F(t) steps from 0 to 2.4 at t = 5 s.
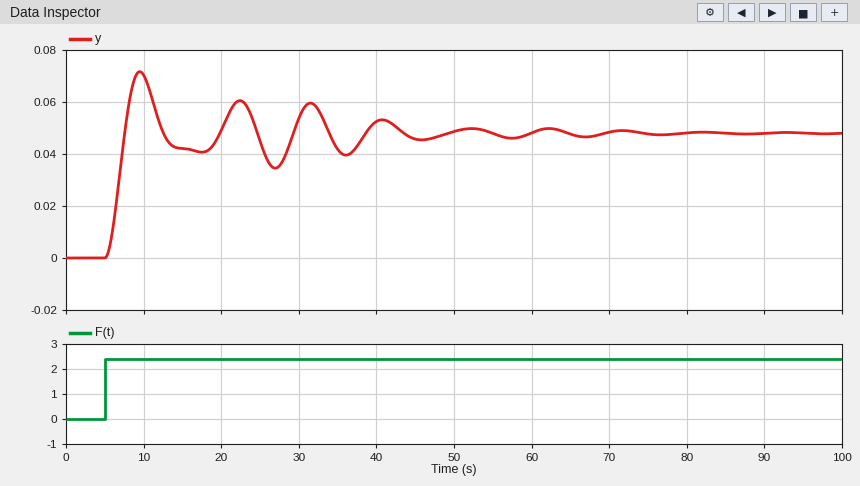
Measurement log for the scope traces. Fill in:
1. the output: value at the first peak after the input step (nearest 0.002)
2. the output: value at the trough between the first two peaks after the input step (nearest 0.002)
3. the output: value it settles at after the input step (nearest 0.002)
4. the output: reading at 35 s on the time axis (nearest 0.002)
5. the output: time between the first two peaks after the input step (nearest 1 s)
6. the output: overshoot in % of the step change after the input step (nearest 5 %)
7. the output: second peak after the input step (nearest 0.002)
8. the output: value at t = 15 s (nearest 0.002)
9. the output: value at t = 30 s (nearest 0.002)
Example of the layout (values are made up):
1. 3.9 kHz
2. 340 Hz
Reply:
1. 0.072
2. 0.040
3. 0.048
4. 0.042
5. 13 s
6. 50 %
7. 0.060
8. 0.042
9. 0.054
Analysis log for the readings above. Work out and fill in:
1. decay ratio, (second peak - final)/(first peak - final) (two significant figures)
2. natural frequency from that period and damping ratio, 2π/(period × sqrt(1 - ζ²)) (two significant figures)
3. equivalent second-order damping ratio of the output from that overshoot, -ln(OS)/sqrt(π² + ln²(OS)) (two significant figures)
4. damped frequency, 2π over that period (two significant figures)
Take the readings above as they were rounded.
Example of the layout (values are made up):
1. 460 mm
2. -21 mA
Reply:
1. 0.50
2. 0.50 rad/s
3. 0.22
4. 0.48 rad/s
